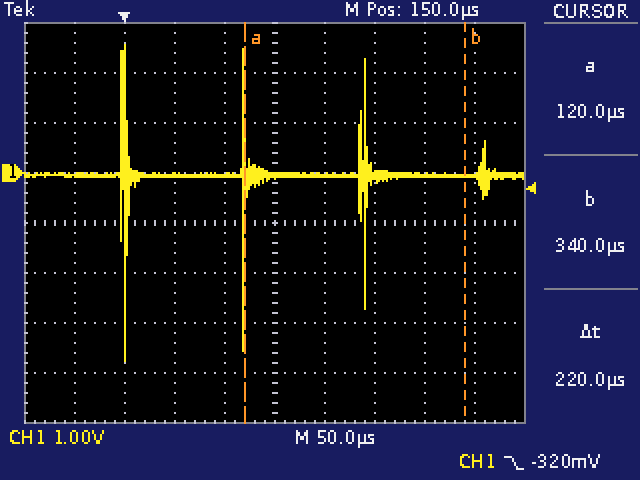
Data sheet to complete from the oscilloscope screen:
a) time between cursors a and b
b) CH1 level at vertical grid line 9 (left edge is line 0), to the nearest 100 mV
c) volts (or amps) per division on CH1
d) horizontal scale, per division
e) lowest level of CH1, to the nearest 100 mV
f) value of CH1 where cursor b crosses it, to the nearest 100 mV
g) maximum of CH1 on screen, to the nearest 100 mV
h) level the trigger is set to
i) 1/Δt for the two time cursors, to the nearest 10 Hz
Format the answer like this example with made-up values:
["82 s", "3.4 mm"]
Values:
["220 µs", "-100 mV", "1 V", "50 µs", "-3.8 V", "-100 mV", "2.6 V", "-320 mV", "4.55 kHz"]
